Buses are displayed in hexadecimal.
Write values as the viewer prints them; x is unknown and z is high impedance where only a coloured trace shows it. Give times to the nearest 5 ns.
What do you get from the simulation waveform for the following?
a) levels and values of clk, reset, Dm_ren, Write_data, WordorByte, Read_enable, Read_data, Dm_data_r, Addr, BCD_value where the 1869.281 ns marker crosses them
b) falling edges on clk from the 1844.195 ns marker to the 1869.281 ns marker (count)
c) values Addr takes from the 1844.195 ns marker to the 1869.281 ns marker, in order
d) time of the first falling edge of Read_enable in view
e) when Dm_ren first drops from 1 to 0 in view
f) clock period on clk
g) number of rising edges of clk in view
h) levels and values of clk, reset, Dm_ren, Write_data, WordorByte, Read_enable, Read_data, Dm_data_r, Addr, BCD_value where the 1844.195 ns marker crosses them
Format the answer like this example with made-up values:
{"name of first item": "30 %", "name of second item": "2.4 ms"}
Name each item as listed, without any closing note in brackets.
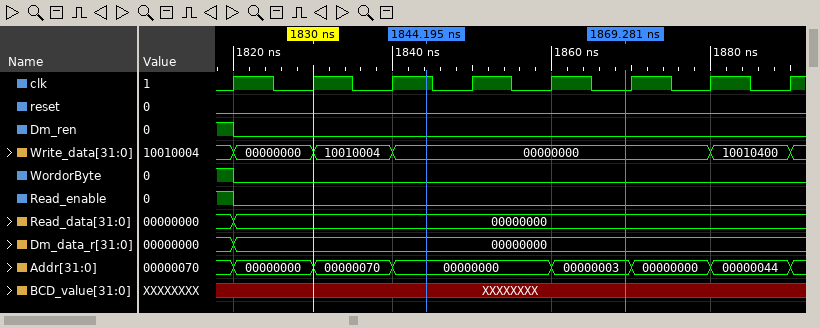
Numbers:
{"levels and values of clk, reset, Dm_ren, Write_data, WordorByte, Read_enable, Read_data, Dm_data_r, Addr, BCD_value where the 1869.281 ns marker crosses them": "clk=0, reset=0, Dm_ren=0, Write_data=00000000, WordorByte=0, Read_enable=0, Read_data=00000000, Dm_data_r=00000000, Addr=00000003, BCD_value=XXXXXXXX", "falling edges on clk from the 1844.195 ns marker to the 1869.281 ns marker": "3", "values Addr takes from the 1844.195 ns marker to the 1869.281 ns marker, in order": "00000000, 00000003", "time of the first falling edge of Read_enable in view": "1820 ns", "when Dm_ren first drops from 1 to 0 in view": "1820 ns", "clock period on clk": "10 ns", "number of rising edges of clk in view": "8", "levels and values of clk, reset, Dm_ren, Write_data, WordorByte, Read_enable, Read_data, Dm_data_r, Addr, BCD_value where the 1844.195 ns marker crosses them": "clk=1, reset=0, Dm_ren=0, Write_data=00000000, WordorByte=0, Read_enable=0, Read_data=00000000, Dm_data_r=00000000, Addr=00000000, BCD_value=XXXXXXXX"}
